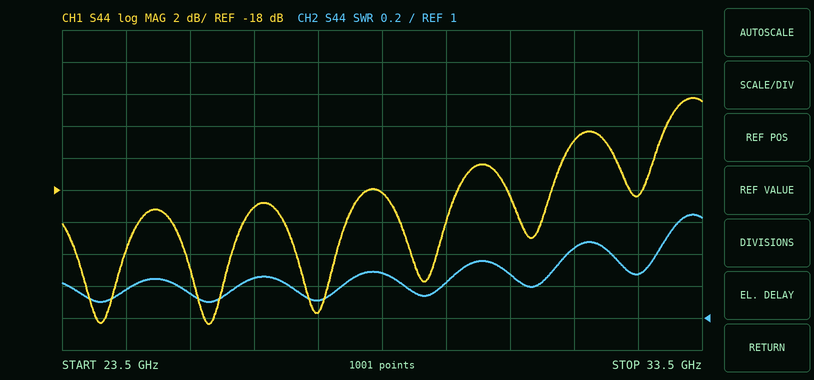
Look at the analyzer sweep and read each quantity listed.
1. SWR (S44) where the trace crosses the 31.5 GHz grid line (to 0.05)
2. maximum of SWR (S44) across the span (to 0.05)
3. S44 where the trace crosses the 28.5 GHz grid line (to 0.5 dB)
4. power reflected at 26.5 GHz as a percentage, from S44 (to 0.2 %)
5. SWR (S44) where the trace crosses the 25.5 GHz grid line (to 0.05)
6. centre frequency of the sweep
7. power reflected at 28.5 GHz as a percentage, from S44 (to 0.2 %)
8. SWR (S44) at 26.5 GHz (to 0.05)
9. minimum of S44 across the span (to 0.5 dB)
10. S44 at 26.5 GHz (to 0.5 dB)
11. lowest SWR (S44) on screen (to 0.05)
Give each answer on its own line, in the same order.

1.45
1.65
-18.0 dB
1.2 %
1.15
28.5 GHz
1.6 %
1.25
-26.5 dB
-19.0 dB
1.10
